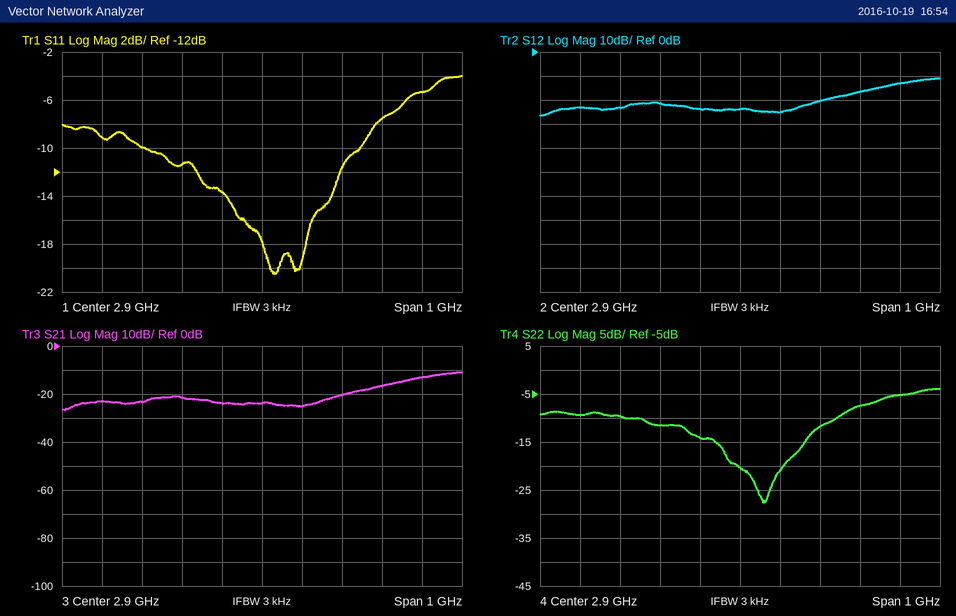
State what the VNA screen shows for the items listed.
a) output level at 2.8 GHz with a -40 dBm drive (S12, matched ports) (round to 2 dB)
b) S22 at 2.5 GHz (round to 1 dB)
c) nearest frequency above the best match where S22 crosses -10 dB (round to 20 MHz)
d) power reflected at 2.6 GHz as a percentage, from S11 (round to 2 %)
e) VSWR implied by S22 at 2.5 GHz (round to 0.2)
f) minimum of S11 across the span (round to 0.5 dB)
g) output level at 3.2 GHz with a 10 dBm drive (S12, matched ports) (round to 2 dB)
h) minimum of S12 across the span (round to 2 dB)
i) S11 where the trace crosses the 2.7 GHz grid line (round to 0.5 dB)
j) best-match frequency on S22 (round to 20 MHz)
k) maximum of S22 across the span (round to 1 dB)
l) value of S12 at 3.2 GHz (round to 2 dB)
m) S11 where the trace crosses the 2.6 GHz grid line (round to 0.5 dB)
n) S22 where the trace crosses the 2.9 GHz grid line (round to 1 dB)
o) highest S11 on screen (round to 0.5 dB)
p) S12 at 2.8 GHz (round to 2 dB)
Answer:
-64 dBm
-9 dB
3.14 GHz
10 %
2.0
-20.5 dB
-6 dBm
-26 dB
-11.5 dB
2.96 GHz
-4 dB
-16 dB
-10.0 dB
-20 dB
-4.0 dB
-24 dB
